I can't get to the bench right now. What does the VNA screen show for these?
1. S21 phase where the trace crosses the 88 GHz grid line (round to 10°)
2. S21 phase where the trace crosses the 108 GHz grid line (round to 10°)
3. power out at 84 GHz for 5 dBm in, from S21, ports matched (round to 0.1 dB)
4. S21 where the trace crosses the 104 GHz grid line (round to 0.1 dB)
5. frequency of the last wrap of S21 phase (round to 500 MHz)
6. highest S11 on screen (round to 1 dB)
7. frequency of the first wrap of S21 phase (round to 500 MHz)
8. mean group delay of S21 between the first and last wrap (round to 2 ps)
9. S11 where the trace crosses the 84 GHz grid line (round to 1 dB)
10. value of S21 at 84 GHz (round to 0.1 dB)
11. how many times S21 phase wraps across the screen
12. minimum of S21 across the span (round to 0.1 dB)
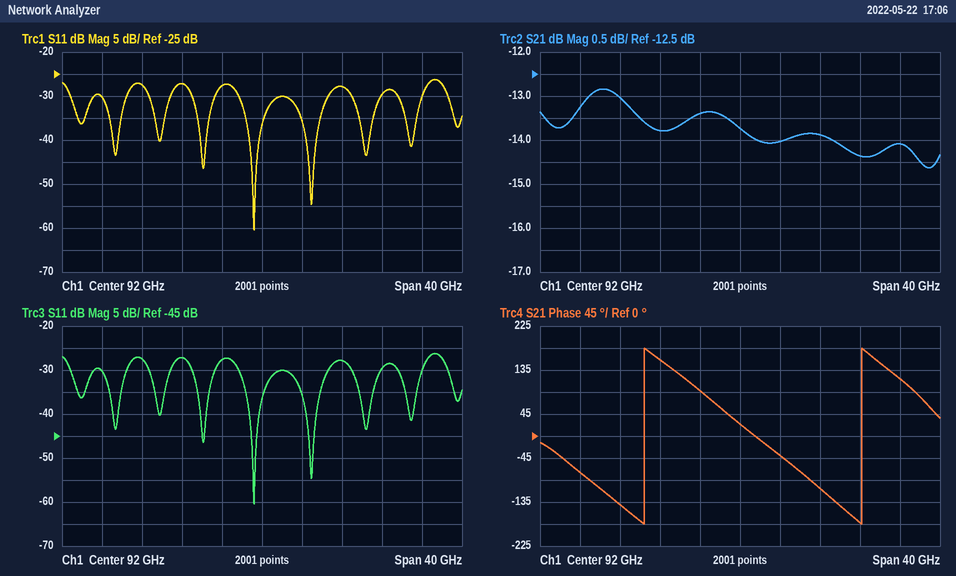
90°
120°
-8.8 dBm
-14.4 dB
104.0 GHz
-26 dB
82.5 GHz
46 ps
-27 dB
-13.8 dB
2
-14.6 dB
